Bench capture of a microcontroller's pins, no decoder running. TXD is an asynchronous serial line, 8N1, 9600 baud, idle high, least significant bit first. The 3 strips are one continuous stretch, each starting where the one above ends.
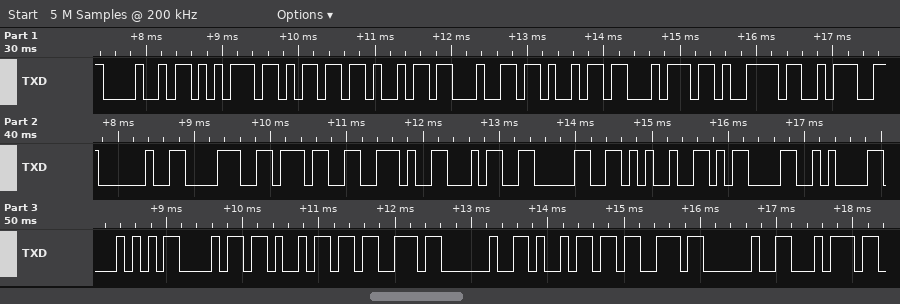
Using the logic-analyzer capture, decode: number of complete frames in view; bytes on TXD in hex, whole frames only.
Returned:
27
0x48 0x75 0x6D 0x69 0x64 0x69 0x74 0x79 0x3A 0x20 0x38 0x37 0x2E 0x34 0x30 0x25 0x0D 0x0A 0x54 0x68 0x69 0x73 0x20 0x69 0x73 0x20 0x74
